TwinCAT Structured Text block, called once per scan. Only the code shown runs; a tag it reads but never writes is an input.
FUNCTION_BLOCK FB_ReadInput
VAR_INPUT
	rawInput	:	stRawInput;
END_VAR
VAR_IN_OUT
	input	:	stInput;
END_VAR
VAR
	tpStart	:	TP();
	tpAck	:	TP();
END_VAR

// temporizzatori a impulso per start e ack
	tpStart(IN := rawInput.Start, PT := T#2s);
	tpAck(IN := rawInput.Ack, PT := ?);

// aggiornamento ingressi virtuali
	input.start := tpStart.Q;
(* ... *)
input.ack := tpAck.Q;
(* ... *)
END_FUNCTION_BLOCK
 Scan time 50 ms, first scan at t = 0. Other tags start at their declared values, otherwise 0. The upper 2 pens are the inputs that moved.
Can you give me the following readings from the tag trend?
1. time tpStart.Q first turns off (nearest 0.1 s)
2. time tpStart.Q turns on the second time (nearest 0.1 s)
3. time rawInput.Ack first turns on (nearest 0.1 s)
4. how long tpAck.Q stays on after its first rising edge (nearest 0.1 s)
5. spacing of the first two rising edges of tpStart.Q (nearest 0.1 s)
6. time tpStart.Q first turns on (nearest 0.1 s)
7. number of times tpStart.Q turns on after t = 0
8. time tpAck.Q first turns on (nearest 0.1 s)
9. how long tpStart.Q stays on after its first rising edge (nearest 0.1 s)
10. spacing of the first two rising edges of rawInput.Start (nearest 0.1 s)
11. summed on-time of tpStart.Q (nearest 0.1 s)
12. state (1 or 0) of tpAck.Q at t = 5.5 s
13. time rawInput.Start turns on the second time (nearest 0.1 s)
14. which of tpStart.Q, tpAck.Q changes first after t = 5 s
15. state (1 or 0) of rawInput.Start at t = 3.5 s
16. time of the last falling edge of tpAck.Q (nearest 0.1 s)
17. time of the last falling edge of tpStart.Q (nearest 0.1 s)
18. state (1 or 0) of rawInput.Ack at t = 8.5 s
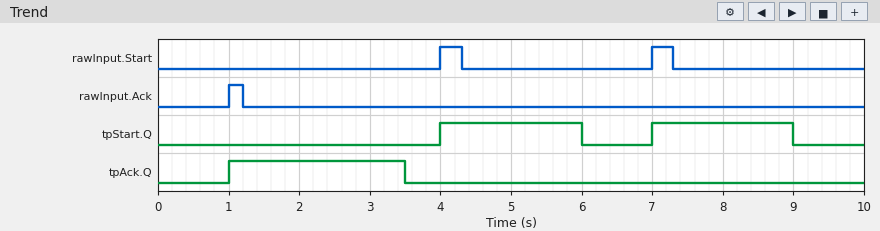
6.0 s
7.0 s
1.0 s
2.5 s
3.0 s
4.0 s
2
1.0 s
2.0 s
3.0 s
4.0 s
0
7.0 s
tpStart.Q
0
3.5 s
9.0 s
0
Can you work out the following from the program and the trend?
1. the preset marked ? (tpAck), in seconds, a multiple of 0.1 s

2.5 s
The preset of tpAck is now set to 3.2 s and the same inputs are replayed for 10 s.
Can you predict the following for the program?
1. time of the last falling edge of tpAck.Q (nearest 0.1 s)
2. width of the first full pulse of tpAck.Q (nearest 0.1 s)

4.2 s
3.2 s
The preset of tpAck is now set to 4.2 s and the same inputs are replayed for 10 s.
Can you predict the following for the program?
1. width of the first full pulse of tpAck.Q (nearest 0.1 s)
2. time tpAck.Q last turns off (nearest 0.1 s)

4.2 s
5.2 s
